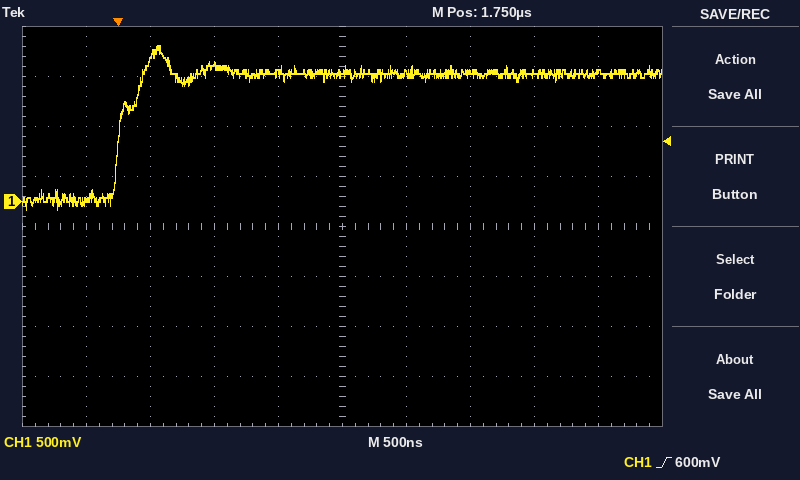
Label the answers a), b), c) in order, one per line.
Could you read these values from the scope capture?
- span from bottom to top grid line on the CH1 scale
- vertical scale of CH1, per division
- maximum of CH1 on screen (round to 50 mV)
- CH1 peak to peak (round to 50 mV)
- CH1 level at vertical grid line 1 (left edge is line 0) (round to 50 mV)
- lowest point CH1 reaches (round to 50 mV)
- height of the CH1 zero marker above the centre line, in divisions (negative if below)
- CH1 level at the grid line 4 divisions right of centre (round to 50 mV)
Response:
a) 4 V
b) 500 mV
c) 1.55 V
d) 1.65 V
e) 0 mV
f) -100 mV
g) +0.5 div
h) 1.30 V
